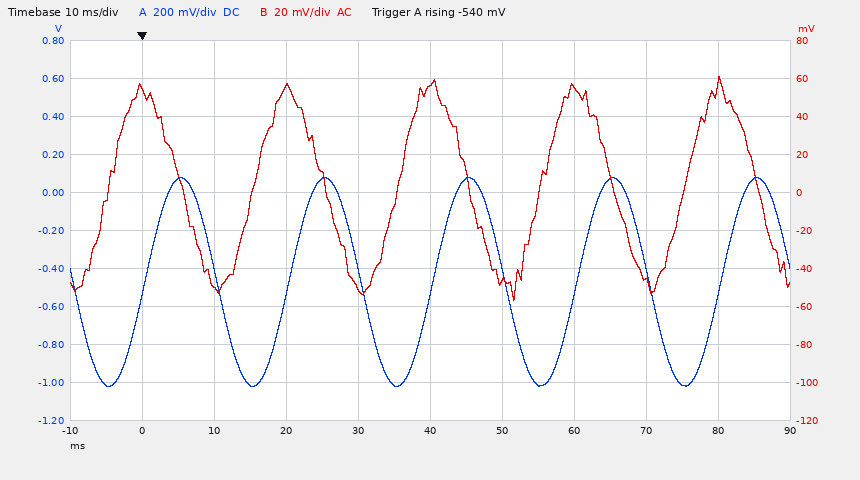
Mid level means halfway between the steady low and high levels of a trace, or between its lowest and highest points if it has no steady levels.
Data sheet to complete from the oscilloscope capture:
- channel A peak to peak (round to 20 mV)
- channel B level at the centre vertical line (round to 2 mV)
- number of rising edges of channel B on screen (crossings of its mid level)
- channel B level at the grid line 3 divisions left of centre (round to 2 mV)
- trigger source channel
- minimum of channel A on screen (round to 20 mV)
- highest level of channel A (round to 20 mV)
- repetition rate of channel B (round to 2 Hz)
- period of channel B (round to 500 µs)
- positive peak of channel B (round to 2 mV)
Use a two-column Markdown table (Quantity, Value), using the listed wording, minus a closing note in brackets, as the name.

| Quantity | Value |
|---|---|
| channel A peak to peak | 1.10 V |
| channel B level at the centre vertical line | 56 mV |
| number of rising edges of channel B on screen | 5 |
| channel B level at the grid line 3 divisions left of centre | -50 mV |
| trigger source channel | channel A |
| minimum of channel A on screen | -1.02 V |
| highest level of channel A | 80 mV |
| repetition rate of channel B | 50 Hz |
| period of channel B | 20.0 ms |
| positive peak of channel B | 62 mV |
